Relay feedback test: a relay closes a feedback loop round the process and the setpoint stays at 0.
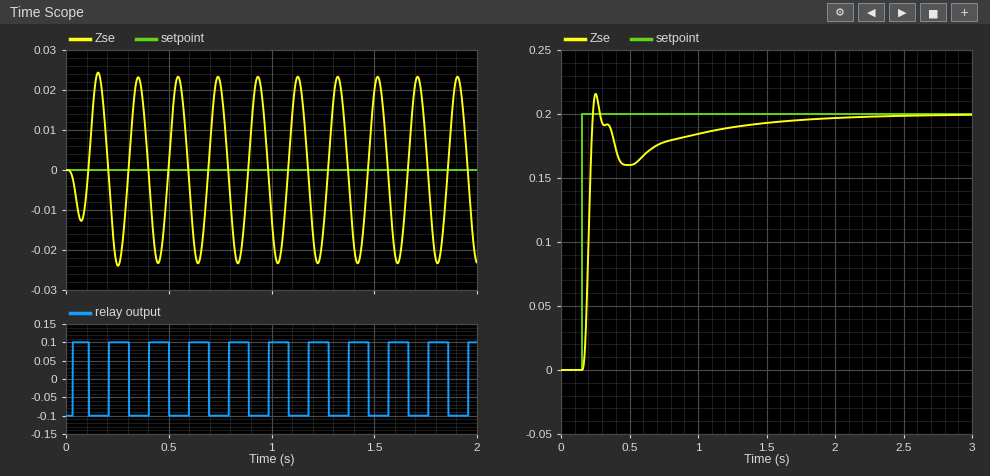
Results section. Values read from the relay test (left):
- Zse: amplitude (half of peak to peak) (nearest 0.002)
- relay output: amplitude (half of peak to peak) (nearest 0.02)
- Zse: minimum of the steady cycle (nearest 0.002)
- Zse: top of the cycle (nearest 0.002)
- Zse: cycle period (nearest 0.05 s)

0.024
0.10
-0.024
0.024
0.20 s
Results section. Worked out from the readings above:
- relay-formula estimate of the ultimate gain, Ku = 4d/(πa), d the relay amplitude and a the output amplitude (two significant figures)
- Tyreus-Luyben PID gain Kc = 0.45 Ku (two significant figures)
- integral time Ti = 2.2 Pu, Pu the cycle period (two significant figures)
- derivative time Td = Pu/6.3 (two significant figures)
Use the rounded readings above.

5.3
2.4
0.44 s
0.032 s
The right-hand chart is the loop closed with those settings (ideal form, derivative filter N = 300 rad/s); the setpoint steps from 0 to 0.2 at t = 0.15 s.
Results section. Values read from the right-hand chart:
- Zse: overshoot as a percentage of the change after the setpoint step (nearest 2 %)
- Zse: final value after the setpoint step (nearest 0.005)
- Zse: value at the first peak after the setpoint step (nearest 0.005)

8 %
0.200
0.215
